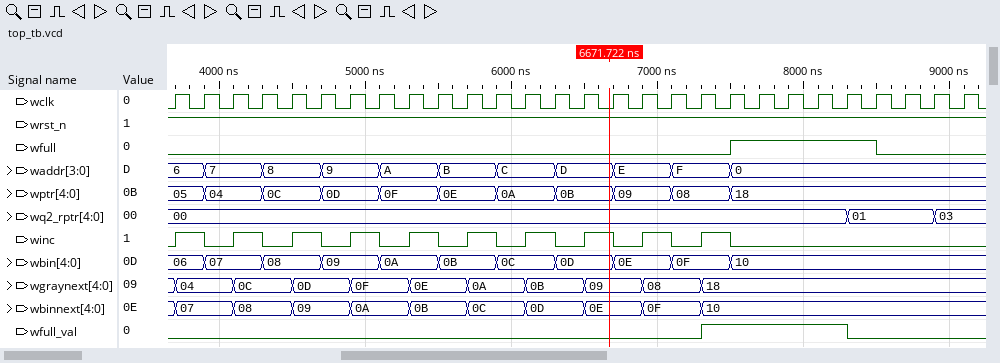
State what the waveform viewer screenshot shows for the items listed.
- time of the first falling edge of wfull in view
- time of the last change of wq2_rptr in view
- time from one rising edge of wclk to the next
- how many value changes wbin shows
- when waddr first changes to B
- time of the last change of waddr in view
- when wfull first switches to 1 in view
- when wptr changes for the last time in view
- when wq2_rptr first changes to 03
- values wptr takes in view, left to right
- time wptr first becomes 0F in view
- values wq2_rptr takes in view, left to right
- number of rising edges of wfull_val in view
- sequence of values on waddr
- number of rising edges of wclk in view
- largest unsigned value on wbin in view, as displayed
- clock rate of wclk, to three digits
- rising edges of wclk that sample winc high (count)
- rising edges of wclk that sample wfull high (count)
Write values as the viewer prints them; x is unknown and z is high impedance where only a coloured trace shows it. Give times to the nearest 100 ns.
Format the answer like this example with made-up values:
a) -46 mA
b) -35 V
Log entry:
a) 8500 ns
b) 8900 ns
c) 200 ns
d) 10
e) 5500 ns
f) 7500 ns
g) 7500 ns
h) 7500 ns
i) 8900 ns
j) 05, 04, 0C, 0D, 0F, 0E, 0A, 0B, 09, 08, 18
k) 5100 ns
l) 00, 01, 03
m) 1
n) 6, 7, 8, 9, A, B, C, D, E, F, 0
o) 28
p) 10
q) 5.00 MHz
r) 10
s) 5
